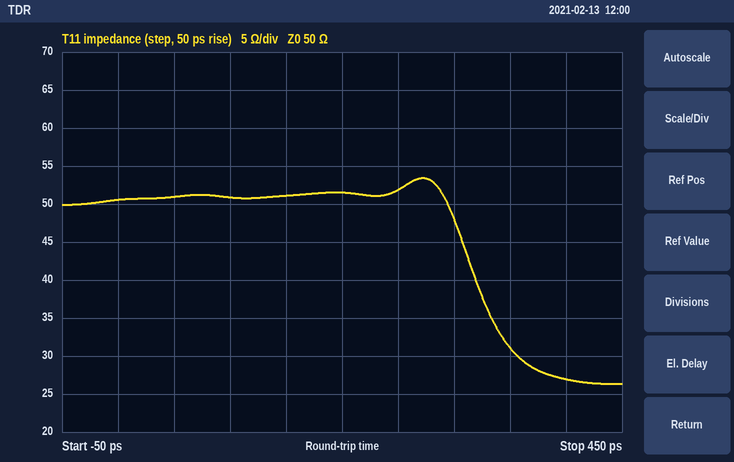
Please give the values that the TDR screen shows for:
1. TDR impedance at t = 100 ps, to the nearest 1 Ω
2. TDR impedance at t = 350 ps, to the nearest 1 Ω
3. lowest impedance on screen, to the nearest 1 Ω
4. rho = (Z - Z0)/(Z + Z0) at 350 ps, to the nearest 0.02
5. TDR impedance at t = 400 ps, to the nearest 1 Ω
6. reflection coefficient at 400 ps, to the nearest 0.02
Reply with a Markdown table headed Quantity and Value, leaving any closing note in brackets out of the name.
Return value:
| Quantity | Value |
|---|---|
| TDR impedance at t = 100 ps, to the nearest 1 Ω | 51 Ω |
| TDR impedance at t = 350 ps, to the nearest 1 Ω | 31 Ω |
| lowest impedance on screen, to the nearest 1 Ω | 26 Ω |
| rho = (Z - Z0)/(Z + Z0) at 350 ps, to the nearest 0.02 | -0.24 |
| TDR impedance at t = 400 ps, to the nearest 1 Ω | 27 Ω |
| reflection coefficient at 400 ps, to the nearest 0.02 | -0.30 |
